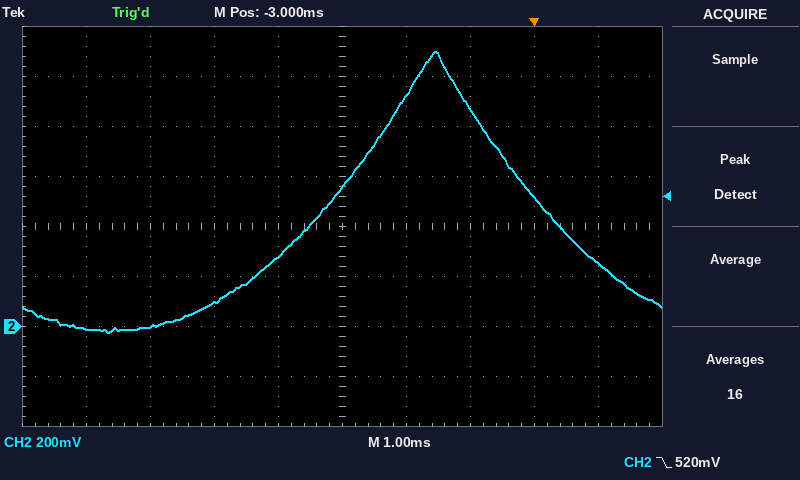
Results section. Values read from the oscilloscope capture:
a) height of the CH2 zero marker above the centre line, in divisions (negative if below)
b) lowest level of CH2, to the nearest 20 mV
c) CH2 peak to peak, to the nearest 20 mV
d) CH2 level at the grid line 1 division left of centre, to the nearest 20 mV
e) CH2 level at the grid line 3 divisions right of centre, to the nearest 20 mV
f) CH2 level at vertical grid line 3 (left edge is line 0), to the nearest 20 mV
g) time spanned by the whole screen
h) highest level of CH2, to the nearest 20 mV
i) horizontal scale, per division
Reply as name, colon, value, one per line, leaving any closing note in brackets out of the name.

height of the CH2 zero marker above the centre line, in divisions: -2.0 div
lowest level of CH2, to the nearest 20 mV: -20 mV
CH2 peak to peak, to the nearest 20 mV: 1.12 V
CH2 level at the grid line 1 division left of centre, to the nearest 20 mV: 280 mV
CH2 level at the grid line 3 divisions right of centre, to the nearest 20 mV: 520 mV
CH2 level at vertical grid line 3 (left edge is line 0), to the nearest 20 mV: 100 mV
time spanned by the whole screen: 10 ms
highest level of CH2, to the nearest 20 mV: 1.10 V
horizontal scale, per division: 1 ms
